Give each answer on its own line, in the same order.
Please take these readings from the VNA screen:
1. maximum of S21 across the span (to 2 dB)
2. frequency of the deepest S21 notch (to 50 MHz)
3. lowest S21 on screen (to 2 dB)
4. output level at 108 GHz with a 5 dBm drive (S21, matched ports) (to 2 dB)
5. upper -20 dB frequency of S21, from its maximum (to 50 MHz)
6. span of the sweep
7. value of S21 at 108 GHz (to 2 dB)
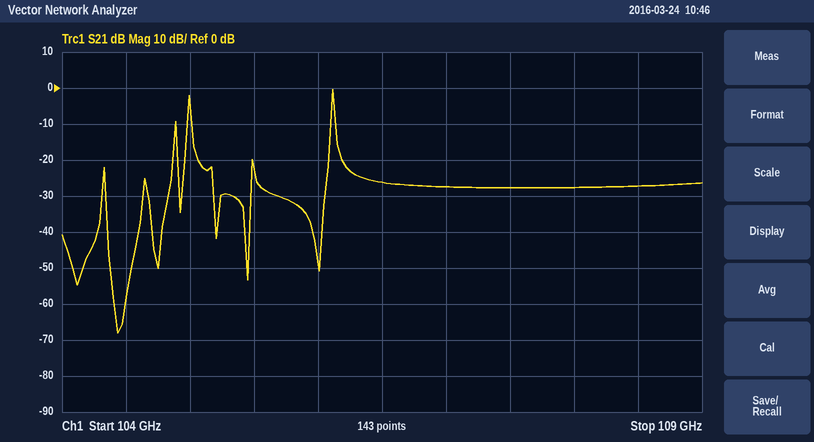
0 dB
104.45 GHz
-68 dB
-22 dBm
106.20 GHz
5 GHz
-28 dB
